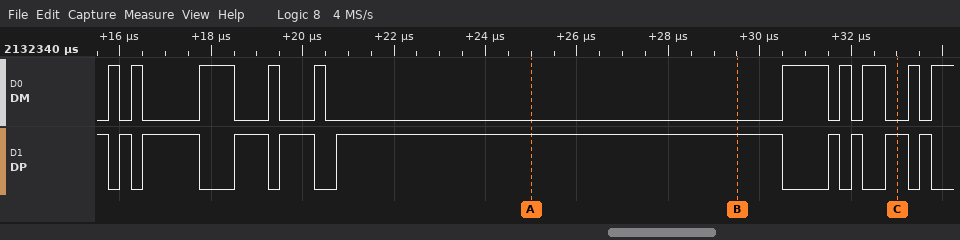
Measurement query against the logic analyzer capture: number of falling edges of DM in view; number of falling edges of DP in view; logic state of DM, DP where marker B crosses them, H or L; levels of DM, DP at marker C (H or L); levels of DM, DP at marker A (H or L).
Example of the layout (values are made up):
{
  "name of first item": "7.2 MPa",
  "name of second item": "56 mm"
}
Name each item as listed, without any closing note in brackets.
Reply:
{
  "number of falling edges of DM in view": "9",
  "number of falling edges of DP in view": "10",
  "logic state of DM, DP where marker B crosses them, H or L": "DM=L, DP=H",
  "levels of DM, DP at marker C": "DM=L, DP=H",
  "levels of DM, DP at marker A": "DM=L, DP=H"
}
